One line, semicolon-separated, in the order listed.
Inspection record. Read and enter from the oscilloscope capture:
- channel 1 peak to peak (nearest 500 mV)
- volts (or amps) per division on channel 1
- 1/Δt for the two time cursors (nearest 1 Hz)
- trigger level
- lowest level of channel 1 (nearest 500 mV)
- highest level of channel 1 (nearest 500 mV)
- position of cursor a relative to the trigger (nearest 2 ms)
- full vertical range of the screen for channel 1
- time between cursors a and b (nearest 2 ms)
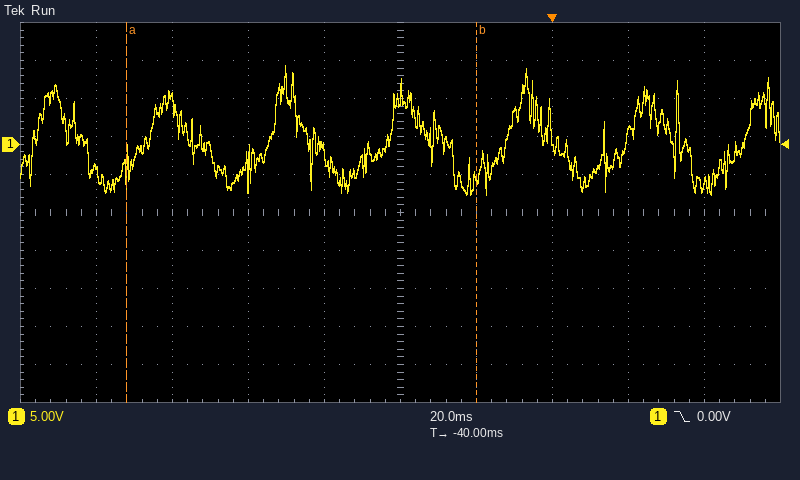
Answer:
17.0 V; 5 V; 11 Hz; 0.00 V; -6.5 V; 10.5 V; -112 ms; 50 V; 92 ms
